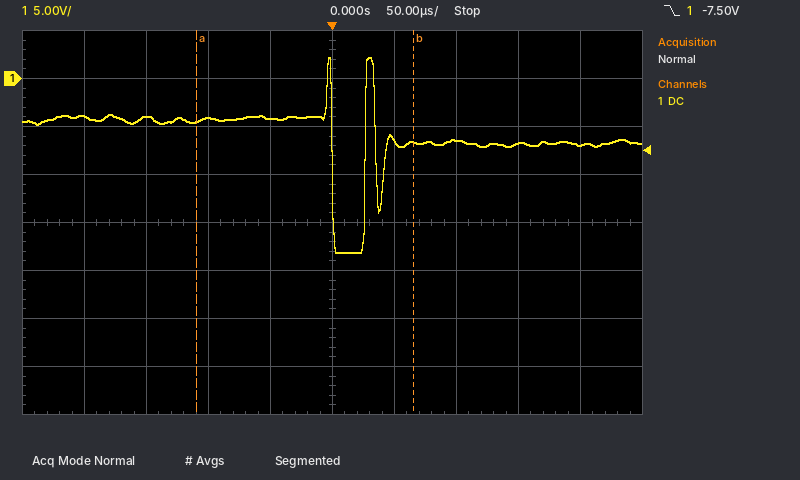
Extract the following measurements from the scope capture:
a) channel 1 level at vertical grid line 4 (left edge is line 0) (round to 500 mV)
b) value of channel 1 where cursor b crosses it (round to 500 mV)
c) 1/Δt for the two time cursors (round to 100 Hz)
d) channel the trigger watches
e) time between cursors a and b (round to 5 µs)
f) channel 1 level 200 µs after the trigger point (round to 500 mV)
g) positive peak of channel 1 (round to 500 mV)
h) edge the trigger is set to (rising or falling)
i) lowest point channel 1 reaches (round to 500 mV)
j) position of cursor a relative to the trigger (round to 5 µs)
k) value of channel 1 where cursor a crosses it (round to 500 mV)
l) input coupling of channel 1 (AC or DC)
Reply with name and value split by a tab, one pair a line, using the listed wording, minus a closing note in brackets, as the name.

channel 1 level at vertical grid line 4 (left edge is line 0)	-4.0 V
value of channel 1 where cursor b crosses it	-6.5 V
1/Δt for the two time cursors	5.7 kHz
channel the trigger watches	channel 1
time between cursors a and b	175 µs
channel 1 level 200 µs after the trigger point	-7.0 V
positive peak of channel 1	2.0 V
edge the trigger is set to	falling
lowest point channel 1 reaches	-18.0 V
position of cursor a relative to the trigger	-110 µs
value of channel 1 where cursor a crosses it	-4.5 V
input coupling of channel 1	DC
